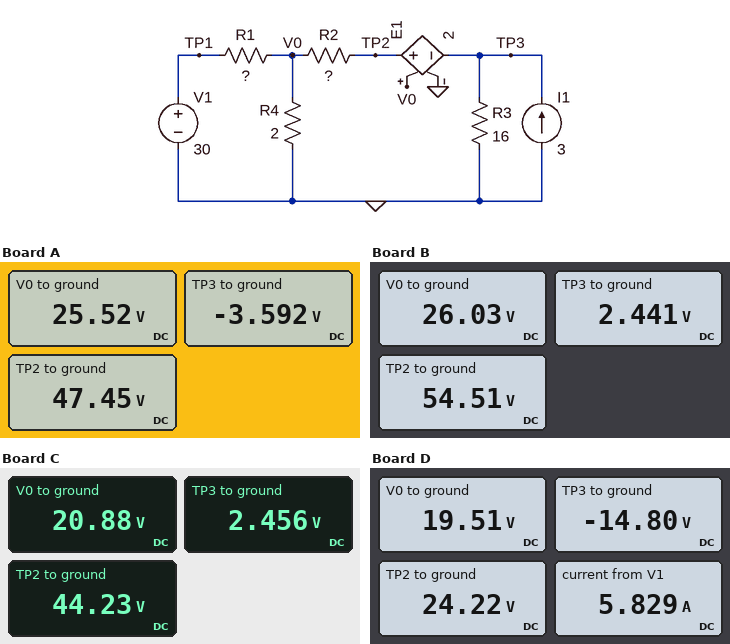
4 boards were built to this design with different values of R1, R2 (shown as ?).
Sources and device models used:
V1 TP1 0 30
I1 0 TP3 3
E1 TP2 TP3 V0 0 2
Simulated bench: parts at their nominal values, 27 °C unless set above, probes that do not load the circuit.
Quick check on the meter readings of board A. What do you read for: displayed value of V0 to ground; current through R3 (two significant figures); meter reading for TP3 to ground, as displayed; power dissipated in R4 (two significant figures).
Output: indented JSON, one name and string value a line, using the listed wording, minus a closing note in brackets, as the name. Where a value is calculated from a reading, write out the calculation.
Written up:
{
  "displayed value of V0 to ground": "25.52 V",
  "current through R3": "(0 V - (-3.592 V)) / 16 Ω = 220 mA",
  "meter reading for TP3 to ground, as displayed": "-3.592 V",
  "power dissipated in R4": "(25.52 V)^2 / 2 Ω = 330 W"
}
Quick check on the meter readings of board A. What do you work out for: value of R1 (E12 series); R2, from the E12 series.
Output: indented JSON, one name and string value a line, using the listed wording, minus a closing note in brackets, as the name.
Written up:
{
  "value of R1": "0.47 Ω",
  "R2, from the E12 series": "6.8 Ω"
}
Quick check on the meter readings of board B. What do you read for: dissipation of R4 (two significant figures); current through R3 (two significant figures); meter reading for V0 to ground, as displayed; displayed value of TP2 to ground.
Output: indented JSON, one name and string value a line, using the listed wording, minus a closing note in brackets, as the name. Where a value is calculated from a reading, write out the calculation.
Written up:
{
  "dissipation of R4": "(26.03 V)^2 / 2 Ω = 340 W",
  "current through R3": "(2.441 V) / 16 Ω = 150 mA",
  "meter reading for V0 to ground, as displayed": "26.03 V",
  "displayed value of TP2 to ground": "54.51 V"
}
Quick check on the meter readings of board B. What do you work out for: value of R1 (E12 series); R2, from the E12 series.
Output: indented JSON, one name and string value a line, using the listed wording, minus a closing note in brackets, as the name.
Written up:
{
  "value of R1": "0.39 Ω",
  "R2, from the E12 series": "10 Ω"
}
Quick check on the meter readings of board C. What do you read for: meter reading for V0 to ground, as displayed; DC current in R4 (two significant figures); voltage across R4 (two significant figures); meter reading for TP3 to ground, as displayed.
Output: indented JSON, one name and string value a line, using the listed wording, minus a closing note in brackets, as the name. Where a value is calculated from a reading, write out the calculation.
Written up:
{
  "meter reading for V0 to ground, as displayed": "20.88 V",
  "DC current in R4": "(20.88 V) / 2 Ω = 10 A",
  "voltage across R4": "20.88 V = 21 V",
  "meter reading for TP3 to ground, as displayed": "2.456 V"
}
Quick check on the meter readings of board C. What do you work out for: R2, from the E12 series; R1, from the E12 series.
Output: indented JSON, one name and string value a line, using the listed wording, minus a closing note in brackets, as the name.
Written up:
{
  "R2, from the E12 series": "8.2 Ω",
  "R1, from the E12 series": "1.2 Ω"
}
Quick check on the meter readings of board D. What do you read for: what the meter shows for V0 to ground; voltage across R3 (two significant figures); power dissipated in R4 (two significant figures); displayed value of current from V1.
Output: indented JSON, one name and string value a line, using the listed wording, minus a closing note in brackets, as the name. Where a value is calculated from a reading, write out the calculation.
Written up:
{
  "what the meter shows for V0 to ground": "19.51 V",
  "voltage across R3": "0 V - (-14.8 V) = 15 V",
  "power dissipated in R4": "(19.51 V)^2 / 2 Ω = 190 W",
  "displayed value of current from V1": "5.829 A"
}
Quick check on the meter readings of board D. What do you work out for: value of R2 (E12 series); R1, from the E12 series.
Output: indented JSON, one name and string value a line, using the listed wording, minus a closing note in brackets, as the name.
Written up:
{
  "value of R2": "1.2 Ω",
  "R1, from the E12 series": "1.8 Ω"
}
